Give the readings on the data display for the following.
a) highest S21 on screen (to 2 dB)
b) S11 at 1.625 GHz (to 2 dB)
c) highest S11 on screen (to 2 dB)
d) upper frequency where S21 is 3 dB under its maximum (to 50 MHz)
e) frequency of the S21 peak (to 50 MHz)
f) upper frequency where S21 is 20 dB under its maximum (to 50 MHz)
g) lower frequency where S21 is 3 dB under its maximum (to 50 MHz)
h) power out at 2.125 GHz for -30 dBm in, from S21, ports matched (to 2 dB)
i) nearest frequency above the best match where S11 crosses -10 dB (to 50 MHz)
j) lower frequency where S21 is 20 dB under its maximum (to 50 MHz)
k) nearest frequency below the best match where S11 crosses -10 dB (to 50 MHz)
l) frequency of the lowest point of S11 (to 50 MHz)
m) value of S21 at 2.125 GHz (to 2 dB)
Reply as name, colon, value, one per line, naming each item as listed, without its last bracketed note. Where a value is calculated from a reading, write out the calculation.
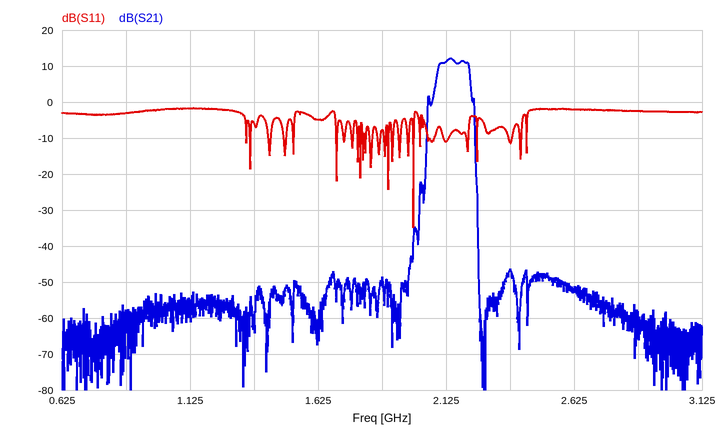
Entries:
highest S21 on screen: 12 dB
S11 at 1.625 GHz: -4 dB
highest S11 on screen: -2 dB
upper frequency where S21 is 3 dB under its maximum: 2.20 GHz
frequency of the S21 peak: 2.15 GHz
upper frequency where S21 is 20 dB under its maximum: 2.25 GHz
lower frequency where S21 is 3 dB under its maximum: 2.10 GHz
power out at 2.125 GHz for -30 dBm in, from S21, ports matched: -30 dBm + (12 dB) = -18 dBm
nearest frequency above the best match where S11 crosses -10 dB: 2.00 GHz
lower frequency where S21 is 20 dB under its maximum: 2.05 GHz
nearest frequency below the best match where S11 crosses -10 dB: 2.00 GHz
frequency of the lowest point of S11: 2.00 GHz
value of S21 at 2.125 GHz: 12 dB
